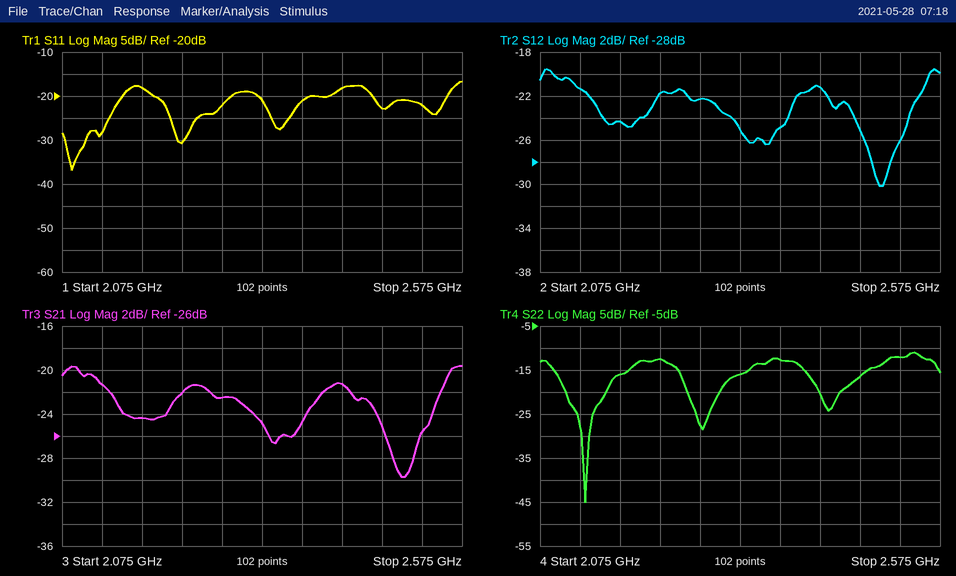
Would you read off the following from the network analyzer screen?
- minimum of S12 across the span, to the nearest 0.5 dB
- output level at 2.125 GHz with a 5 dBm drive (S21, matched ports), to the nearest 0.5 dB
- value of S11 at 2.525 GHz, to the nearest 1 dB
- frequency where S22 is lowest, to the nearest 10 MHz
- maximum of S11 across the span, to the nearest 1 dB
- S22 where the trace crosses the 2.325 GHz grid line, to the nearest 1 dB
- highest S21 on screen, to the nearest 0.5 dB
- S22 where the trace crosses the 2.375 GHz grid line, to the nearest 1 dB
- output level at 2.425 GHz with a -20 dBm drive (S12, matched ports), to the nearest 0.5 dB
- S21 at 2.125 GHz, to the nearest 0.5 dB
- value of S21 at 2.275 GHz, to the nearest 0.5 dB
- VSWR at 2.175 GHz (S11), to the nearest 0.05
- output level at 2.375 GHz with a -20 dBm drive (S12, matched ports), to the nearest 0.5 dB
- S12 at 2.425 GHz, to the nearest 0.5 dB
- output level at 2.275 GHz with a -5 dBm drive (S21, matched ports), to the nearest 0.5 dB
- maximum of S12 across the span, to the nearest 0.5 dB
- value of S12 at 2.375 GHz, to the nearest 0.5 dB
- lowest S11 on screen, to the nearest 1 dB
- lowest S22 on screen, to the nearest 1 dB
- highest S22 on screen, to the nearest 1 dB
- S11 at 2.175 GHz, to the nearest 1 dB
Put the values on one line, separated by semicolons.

-30.0 dB; -16.5 dBm; -22 dB; 2.13 GHz; -17 dB; -16 dB; -19.5 dB; -13 dB; -41.0 dBm; -21.5 dB; -22.5 dB; 1.30; -45.0 dBm; -21.0 dB; -27.5 dBm; -19.5 dB; -25.0 dB; -37 dB; -45 dB; -11 dB; -18 dB
